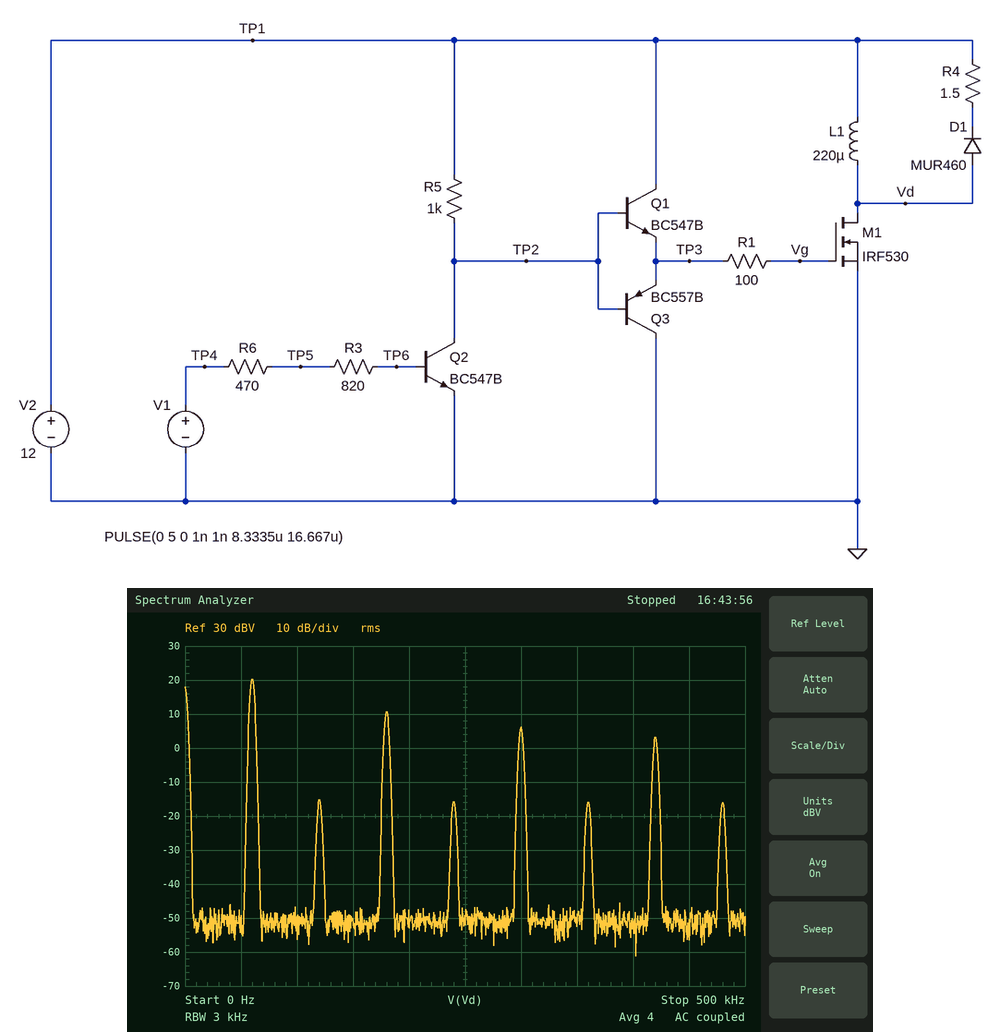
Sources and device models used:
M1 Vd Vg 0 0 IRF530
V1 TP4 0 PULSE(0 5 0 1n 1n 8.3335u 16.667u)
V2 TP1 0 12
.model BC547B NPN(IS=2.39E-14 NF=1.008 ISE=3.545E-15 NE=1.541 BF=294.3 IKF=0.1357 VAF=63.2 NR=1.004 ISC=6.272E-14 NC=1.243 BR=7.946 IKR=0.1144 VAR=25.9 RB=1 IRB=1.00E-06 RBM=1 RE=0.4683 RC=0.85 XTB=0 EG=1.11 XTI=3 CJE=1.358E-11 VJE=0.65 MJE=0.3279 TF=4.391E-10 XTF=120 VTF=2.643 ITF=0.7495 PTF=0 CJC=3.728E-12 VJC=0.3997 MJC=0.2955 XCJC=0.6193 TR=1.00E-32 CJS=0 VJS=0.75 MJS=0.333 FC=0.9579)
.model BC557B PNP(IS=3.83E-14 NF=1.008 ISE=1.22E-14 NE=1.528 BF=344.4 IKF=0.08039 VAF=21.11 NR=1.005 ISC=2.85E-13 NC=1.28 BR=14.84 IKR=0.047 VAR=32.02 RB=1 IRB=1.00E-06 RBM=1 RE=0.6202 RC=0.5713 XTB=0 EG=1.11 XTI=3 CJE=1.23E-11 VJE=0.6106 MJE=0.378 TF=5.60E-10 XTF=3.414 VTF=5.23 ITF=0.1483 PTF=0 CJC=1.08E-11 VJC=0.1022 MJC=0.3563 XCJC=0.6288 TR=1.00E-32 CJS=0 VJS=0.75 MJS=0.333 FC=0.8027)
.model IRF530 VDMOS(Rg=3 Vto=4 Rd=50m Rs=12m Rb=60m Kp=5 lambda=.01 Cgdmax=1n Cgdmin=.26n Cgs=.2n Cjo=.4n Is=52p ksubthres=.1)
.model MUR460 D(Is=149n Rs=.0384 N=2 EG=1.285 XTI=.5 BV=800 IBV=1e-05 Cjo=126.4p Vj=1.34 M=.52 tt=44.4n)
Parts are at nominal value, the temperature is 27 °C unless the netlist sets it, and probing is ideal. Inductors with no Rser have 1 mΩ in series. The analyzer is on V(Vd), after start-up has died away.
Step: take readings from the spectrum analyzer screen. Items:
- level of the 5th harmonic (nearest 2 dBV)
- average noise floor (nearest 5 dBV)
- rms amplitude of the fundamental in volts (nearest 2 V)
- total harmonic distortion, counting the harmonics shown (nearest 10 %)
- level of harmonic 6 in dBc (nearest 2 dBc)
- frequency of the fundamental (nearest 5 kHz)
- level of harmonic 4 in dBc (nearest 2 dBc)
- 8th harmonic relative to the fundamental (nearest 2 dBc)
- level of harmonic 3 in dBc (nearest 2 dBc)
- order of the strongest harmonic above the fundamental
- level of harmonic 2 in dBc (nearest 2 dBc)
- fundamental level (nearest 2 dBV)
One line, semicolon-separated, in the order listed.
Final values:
6 dBV; -50 dBV; 10 V; 40 %; -36 dBc; 60 kHz; -36 dBc; -36 dBc; -10 dBc; 3; -36 dBc; 20 dBV
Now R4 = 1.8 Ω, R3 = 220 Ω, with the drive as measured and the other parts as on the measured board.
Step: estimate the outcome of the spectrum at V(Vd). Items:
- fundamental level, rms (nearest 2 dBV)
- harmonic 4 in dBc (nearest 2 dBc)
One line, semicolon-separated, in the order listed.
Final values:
20 dBV; -34 dBc
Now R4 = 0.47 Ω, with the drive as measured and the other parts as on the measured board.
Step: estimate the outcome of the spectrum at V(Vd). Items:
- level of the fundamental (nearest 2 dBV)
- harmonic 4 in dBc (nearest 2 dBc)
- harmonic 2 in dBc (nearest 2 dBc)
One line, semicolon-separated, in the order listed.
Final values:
20 dBV; -56 dBc; -52 dBc
